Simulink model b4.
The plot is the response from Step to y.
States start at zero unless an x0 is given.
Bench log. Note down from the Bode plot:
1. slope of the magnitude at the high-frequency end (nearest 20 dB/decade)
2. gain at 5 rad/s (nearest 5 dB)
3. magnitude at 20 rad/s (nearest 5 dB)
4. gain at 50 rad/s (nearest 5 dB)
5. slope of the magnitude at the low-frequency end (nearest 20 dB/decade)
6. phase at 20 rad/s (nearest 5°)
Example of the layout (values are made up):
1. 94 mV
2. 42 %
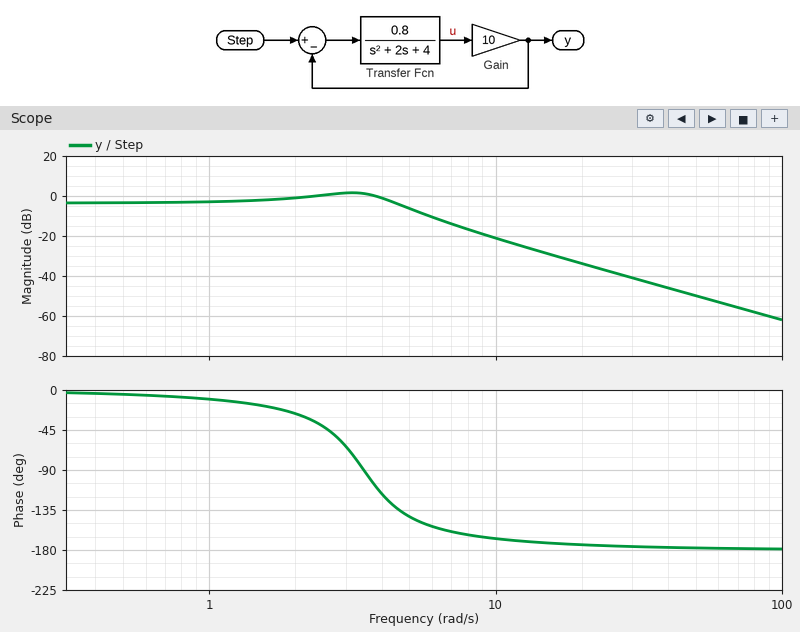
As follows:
1. -40 dB/decade
2. -5 dB
3. -35 dB
4. -50 dB
5. 0 dB/decade
6. -175°
